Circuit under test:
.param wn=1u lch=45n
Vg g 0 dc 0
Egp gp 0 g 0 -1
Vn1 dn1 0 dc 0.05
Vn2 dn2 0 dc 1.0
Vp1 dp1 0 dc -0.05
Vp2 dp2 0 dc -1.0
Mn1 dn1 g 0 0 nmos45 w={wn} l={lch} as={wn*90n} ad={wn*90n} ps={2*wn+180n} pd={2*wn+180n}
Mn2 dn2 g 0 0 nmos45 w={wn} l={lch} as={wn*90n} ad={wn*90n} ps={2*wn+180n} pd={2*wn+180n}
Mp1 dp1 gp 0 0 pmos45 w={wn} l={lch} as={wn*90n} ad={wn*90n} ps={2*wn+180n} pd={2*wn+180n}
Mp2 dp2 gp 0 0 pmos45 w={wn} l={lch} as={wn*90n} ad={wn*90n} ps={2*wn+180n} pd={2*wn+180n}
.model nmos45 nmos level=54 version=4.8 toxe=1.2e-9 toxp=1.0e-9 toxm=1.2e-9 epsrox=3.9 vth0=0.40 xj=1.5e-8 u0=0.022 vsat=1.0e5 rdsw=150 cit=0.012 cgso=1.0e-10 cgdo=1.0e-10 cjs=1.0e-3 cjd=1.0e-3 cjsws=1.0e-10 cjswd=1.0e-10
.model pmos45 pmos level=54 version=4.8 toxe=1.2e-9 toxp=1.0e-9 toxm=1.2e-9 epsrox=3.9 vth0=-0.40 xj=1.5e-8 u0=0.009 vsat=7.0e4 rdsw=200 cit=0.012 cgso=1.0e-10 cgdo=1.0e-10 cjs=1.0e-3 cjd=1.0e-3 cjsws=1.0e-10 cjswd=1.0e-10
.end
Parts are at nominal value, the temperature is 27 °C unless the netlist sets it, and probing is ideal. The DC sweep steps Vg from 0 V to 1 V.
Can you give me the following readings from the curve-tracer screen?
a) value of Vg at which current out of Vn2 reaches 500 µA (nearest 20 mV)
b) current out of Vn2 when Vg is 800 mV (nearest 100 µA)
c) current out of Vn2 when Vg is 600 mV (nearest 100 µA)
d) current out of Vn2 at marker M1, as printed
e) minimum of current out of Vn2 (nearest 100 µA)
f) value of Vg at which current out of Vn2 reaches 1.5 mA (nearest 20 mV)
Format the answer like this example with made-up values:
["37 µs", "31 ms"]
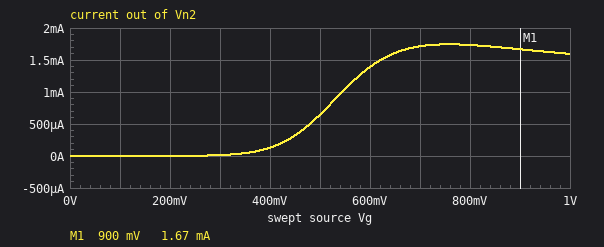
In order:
["480 mV", "1.7 mA", "1.4 mA", "1.67 mA", "0 A", "620 mV"]
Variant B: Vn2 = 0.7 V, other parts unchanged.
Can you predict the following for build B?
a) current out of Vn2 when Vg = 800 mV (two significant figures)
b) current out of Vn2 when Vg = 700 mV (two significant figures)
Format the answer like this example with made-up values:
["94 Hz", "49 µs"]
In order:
["530 µA", "390 µA"]
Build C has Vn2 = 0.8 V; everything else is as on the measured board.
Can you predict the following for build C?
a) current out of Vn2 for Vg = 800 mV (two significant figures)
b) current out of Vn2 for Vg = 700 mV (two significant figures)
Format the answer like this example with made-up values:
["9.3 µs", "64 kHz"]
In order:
["670 µA", "570 µA"]
